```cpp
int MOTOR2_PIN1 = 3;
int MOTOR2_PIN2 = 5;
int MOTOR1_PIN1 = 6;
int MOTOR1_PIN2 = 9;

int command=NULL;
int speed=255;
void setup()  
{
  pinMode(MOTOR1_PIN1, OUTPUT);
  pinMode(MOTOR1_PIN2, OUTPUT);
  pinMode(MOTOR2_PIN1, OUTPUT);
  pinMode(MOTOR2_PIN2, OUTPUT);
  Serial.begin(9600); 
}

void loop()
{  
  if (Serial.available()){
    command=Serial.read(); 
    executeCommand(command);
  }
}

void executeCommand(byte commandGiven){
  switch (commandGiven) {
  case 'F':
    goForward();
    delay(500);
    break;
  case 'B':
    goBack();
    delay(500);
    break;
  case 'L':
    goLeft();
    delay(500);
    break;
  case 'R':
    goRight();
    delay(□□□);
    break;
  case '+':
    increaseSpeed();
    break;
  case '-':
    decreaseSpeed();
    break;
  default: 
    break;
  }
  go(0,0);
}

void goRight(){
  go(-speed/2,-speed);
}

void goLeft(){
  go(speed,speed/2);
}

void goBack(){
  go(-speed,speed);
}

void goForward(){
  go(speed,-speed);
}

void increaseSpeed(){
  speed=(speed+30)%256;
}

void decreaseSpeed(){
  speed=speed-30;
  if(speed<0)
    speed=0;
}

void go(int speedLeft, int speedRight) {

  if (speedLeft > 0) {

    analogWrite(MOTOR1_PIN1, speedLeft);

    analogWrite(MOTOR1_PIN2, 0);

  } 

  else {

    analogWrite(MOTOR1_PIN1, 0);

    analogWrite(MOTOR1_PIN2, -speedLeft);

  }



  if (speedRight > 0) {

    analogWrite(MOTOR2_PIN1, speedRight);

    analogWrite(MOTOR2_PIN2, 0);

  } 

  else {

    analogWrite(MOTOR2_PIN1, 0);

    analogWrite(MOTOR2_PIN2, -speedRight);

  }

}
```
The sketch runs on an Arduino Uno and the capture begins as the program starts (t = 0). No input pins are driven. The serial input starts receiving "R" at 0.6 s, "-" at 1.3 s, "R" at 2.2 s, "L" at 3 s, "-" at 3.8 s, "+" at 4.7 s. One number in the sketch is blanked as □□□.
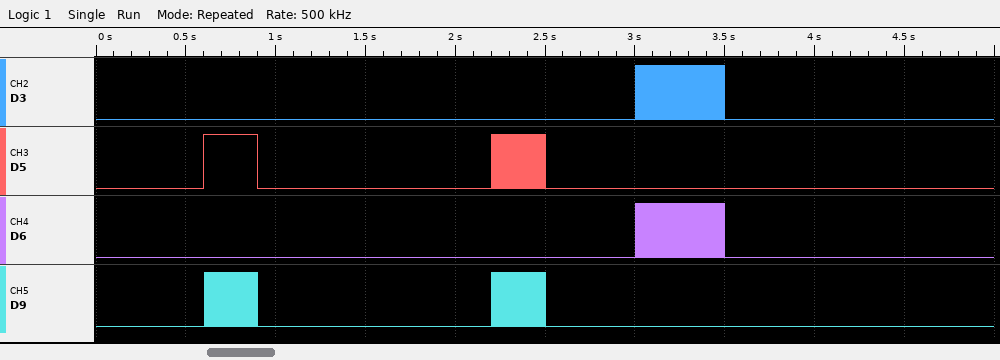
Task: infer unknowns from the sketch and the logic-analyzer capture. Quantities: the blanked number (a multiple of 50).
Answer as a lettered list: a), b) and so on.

a) 300
